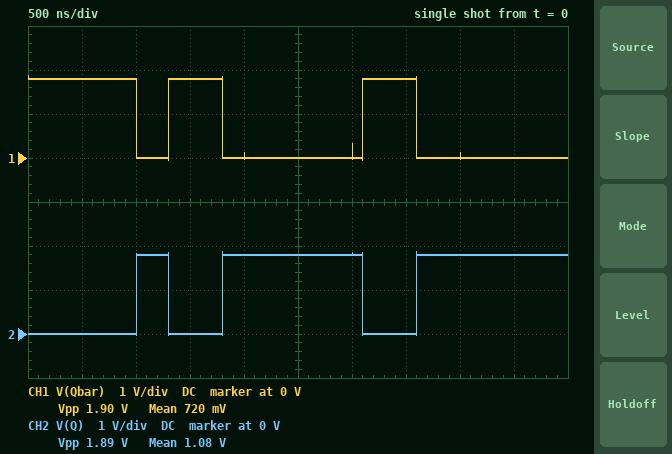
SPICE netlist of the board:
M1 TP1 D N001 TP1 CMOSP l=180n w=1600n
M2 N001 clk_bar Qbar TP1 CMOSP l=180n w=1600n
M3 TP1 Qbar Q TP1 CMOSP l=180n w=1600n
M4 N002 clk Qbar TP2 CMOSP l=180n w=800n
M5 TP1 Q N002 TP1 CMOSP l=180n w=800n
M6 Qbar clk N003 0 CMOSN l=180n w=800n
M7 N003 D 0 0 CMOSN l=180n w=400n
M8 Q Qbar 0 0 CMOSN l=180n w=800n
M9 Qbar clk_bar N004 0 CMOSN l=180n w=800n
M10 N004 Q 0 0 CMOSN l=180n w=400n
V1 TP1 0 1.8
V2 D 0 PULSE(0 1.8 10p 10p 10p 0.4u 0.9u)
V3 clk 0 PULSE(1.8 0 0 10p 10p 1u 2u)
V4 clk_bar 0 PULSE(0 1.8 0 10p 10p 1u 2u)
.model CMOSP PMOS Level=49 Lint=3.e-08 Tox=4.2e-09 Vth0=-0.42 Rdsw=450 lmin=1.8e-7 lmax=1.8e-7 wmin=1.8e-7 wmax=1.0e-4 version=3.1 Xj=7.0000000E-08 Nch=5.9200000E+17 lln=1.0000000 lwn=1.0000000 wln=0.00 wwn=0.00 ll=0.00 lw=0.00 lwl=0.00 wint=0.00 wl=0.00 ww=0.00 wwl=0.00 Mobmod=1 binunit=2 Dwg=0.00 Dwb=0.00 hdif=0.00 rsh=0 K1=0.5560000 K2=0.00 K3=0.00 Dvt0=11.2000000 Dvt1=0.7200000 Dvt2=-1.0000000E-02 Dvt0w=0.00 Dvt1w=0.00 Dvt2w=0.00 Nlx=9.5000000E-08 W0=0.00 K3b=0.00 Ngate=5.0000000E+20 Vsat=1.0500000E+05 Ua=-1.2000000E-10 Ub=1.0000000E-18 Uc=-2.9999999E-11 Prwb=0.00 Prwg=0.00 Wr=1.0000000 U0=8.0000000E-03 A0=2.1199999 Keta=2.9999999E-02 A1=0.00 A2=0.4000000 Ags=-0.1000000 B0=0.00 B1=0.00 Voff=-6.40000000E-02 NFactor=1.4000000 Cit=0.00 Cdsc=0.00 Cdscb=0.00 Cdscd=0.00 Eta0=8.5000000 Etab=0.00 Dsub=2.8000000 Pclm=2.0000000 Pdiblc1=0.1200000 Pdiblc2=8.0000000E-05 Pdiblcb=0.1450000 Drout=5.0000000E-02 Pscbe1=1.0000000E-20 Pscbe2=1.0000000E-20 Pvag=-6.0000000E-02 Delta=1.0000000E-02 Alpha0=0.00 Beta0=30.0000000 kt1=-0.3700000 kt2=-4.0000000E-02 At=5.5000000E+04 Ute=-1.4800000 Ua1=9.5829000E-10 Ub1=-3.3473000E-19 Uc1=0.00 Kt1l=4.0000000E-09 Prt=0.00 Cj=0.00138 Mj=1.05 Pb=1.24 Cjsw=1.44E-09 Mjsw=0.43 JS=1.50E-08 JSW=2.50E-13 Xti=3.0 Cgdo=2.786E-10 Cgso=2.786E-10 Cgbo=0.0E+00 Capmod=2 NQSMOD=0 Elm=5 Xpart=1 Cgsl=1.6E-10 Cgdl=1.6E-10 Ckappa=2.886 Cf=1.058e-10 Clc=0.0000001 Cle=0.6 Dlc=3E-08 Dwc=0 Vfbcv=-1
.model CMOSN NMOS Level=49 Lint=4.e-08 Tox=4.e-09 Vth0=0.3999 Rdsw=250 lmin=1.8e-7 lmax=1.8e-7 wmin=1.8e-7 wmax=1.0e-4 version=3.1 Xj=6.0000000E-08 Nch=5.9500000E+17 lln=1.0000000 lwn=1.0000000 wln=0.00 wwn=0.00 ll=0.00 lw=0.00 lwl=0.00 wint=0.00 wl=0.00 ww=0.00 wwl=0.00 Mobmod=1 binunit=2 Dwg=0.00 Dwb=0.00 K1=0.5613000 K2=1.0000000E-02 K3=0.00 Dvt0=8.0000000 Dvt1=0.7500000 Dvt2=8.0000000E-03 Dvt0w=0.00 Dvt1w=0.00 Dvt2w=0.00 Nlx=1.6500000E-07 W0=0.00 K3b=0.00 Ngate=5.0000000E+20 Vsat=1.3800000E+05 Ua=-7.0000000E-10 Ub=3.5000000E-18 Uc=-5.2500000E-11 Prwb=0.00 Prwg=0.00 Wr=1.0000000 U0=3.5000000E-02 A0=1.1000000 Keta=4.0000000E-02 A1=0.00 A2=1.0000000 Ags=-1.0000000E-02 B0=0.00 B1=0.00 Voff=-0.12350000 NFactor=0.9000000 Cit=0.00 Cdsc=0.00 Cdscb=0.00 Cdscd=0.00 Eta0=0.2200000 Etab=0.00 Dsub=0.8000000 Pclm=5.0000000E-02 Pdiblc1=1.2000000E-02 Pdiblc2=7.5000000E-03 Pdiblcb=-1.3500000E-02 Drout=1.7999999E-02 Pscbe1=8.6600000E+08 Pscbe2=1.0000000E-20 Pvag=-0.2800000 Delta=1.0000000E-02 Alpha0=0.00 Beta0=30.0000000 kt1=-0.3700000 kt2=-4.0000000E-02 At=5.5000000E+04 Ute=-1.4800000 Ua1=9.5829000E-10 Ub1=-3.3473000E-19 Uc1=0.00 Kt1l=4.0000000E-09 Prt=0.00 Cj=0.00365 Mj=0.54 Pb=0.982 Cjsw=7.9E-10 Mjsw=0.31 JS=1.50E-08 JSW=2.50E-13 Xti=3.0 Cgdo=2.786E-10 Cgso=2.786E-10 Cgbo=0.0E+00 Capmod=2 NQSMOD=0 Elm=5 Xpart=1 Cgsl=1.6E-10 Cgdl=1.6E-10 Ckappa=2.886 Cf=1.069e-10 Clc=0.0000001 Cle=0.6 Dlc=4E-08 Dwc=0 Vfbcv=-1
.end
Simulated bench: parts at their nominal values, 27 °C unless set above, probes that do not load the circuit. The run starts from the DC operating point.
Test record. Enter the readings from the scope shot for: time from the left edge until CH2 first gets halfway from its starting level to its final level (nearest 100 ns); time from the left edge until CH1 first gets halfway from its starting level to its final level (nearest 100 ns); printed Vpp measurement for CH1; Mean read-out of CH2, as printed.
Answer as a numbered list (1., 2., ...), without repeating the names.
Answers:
1. 1.0 µs
2. 1.0 µs
3. 1.90 V
4. 1.08 V
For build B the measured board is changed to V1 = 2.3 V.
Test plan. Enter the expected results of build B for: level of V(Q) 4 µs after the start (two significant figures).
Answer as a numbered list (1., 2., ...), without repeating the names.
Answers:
1. 2.3 V
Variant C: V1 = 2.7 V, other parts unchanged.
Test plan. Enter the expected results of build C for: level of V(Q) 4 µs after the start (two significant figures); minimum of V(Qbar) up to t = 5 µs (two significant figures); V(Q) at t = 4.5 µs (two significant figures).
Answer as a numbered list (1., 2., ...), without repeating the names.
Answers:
1. 2.6 V
2. 170 mV
3. 2.7 V
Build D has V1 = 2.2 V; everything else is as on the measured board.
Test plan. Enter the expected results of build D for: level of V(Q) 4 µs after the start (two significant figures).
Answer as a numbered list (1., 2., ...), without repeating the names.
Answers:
1. 2.2 V
